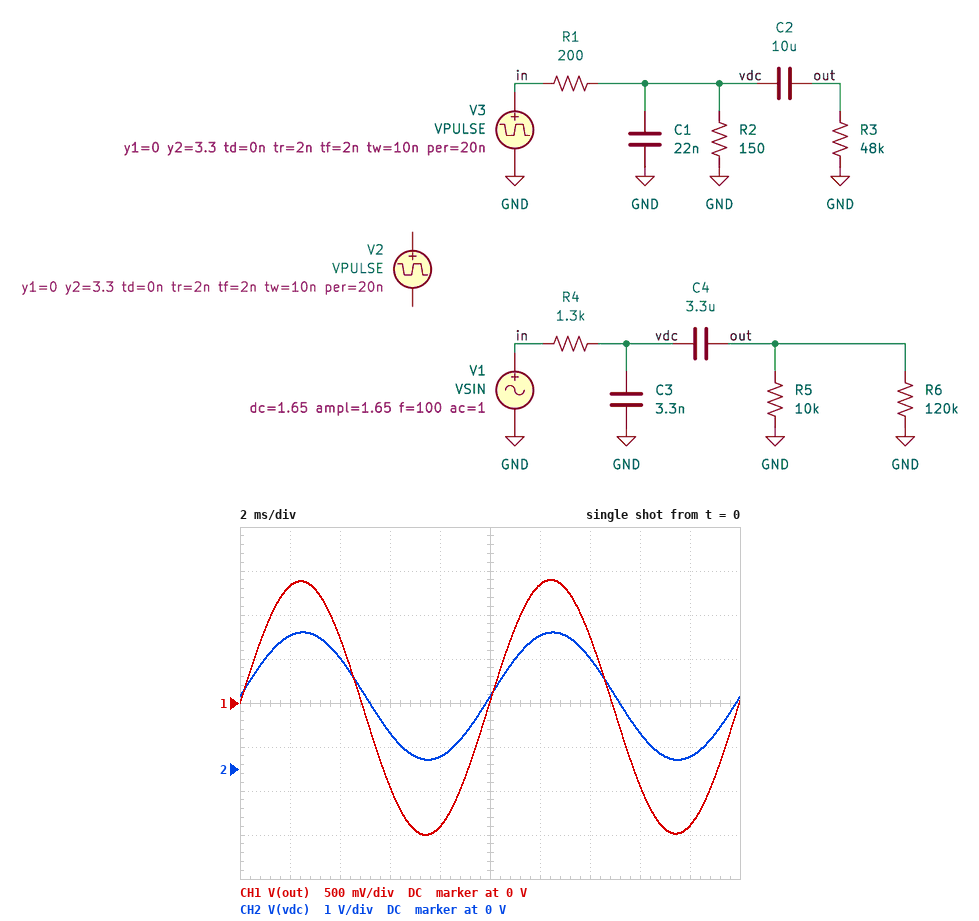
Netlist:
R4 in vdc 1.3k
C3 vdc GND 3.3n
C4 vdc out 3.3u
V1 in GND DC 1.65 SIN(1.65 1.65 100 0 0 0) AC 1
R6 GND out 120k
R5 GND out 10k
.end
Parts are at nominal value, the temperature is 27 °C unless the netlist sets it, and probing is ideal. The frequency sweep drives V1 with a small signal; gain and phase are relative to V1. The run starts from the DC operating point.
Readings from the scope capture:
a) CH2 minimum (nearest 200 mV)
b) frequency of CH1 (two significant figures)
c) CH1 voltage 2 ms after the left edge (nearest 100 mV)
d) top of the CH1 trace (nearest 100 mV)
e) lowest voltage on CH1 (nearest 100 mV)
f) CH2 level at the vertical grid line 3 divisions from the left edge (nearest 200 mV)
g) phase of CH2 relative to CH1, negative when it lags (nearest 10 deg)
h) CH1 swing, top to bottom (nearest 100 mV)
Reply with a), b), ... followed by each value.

a) 200 mV
b) 100 Hz
c) 1.3 V
d) 1.4 V
e) -1.5 V
f) 800 mV
g) 0 deg
h) 2.9 V
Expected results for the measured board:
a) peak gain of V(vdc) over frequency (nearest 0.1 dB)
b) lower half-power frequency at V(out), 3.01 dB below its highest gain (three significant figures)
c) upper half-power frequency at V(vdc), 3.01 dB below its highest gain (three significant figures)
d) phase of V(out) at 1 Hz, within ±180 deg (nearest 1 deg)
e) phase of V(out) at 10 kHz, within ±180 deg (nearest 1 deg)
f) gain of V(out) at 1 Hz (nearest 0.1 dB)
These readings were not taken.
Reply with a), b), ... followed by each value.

a) 0 dB
b) 4.58 Hz
c) 31.0 kHz
d) 78 deg
e) -13 deg
f) -14.6 dB
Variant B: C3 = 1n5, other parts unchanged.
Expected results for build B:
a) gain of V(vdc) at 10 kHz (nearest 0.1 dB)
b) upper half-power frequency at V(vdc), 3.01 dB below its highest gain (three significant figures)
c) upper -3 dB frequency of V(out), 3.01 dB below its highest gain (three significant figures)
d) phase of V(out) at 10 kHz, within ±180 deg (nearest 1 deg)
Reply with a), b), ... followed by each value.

a) -1.2 dB
b) 68.2 kHz
c) 93.1 kHz
d) -6 deg
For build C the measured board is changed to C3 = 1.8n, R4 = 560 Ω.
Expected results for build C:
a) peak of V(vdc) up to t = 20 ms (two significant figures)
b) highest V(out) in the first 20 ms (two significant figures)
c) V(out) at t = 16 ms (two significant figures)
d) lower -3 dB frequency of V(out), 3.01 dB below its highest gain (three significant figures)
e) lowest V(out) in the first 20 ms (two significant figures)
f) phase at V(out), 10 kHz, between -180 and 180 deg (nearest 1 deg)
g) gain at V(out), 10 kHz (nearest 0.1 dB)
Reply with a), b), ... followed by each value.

a) 3.2 V
b) 1.5 V
c) -1.0 V
d) 4.93 Hz
e) -1.6 V
f) -3 deg
g) -0.5 dB
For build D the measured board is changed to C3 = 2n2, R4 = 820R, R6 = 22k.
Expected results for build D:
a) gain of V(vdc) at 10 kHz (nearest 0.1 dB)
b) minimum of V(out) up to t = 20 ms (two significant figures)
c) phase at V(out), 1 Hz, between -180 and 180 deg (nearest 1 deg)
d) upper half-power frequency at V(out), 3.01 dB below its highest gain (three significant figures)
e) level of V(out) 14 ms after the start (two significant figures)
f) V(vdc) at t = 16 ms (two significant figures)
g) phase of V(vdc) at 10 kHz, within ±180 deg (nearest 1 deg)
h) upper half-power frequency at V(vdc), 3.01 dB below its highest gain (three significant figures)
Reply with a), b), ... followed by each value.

a) -1.0 dB
b) -1.5 V
c) 81 deg
d) 98.8 kHz
e) 740 mV
f) 800 mV
g) -6 deg
h) 76.3 kHz
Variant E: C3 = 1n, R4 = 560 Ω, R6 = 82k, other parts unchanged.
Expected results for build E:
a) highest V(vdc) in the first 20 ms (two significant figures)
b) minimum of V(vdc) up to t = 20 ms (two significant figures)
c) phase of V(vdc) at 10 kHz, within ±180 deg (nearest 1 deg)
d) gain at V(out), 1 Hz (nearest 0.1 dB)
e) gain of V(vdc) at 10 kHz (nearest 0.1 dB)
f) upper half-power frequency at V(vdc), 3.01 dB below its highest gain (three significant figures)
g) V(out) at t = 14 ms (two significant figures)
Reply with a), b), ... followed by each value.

a) 3.2 V
b) 100 mV
c) -2 deg
d) -14.8 dB
e) -0.5 dB
f) 265 kHz
g) 800 mV
